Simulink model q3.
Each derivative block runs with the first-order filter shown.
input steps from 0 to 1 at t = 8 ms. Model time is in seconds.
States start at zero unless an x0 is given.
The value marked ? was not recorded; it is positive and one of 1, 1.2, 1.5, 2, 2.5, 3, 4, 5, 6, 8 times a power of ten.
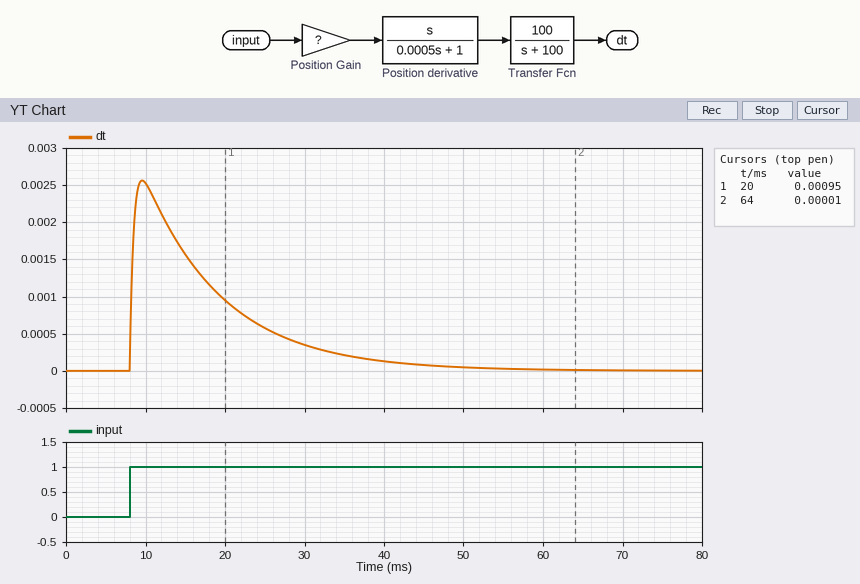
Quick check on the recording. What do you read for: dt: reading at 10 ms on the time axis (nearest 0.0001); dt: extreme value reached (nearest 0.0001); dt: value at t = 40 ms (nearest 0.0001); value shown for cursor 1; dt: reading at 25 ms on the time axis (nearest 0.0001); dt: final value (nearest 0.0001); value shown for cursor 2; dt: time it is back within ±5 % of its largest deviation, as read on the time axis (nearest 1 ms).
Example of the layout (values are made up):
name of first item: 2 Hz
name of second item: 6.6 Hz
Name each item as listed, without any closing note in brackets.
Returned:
dt: reading at 10 ms on the time axis: 0.0025
dt: extreme value reached: 0.0026
dt: value at t = 40 ms: 0.0001
value shown for cursor 1: 0.00095
dt: reading at 25 ms on the time axis: 0.0006
dt: final value: 0.0000
value shown for cursor 2: 0.00001
dt: time it is back within ±5 % of its largest deviation, as read on the time axis: 40 ms
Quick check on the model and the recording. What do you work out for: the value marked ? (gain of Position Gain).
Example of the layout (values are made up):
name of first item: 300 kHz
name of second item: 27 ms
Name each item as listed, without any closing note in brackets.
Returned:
the value marked ?: 3e-05
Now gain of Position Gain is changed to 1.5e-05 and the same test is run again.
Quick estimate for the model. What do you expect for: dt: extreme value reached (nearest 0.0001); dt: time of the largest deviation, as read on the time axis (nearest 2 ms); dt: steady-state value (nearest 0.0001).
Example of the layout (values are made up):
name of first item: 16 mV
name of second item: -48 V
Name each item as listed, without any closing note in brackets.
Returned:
dt: extreme value reached: 0.0013
dt: time of the largest deviation, as read on the time axis: 10 ms
dt: steady-state value: 0.0000
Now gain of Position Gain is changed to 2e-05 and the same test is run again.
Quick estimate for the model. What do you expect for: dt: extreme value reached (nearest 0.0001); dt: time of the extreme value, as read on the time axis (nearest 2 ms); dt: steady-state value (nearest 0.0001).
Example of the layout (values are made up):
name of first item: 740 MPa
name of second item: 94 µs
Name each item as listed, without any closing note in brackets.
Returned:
dt: extreme value reached: 0.0017
dt: time of the extreme value, as read on the time axis: 10 ms
dt: steady-state value: 0.0000
